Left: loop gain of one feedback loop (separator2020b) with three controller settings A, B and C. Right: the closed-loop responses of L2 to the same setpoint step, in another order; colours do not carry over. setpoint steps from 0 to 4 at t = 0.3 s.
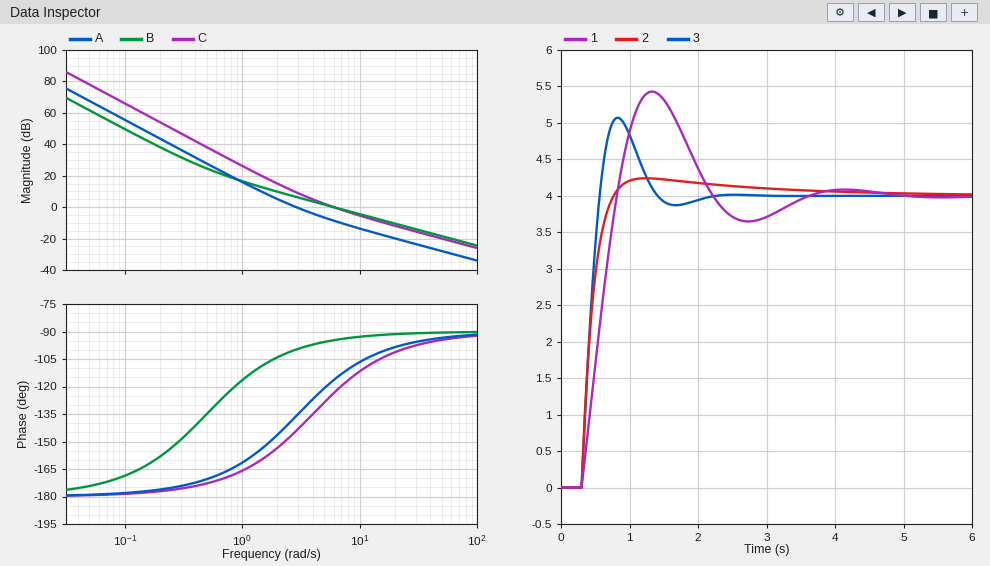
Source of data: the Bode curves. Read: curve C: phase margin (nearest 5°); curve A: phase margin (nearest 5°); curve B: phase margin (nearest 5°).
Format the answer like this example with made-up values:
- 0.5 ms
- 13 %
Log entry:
- 55°
- 45°
- 85°
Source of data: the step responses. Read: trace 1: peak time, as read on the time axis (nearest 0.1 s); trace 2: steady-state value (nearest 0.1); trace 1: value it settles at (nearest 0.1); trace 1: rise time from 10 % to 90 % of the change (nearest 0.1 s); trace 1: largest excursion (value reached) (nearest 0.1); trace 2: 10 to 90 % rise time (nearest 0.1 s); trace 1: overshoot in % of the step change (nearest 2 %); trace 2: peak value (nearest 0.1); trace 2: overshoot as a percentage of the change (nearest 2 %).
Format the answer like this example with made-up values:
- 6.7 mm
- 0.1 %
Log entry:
- 1.3 s
- 4.0
- 4.0
- 0.4 s
- 5.4
- 0.3 s
- 36 %
- 4.2
- 6 %
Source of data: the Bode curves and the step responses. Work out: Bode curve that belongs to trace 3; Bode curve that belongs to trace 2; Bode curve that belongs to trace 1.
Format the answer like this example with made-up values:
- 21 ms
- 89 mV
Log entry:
- C
- B
- A
